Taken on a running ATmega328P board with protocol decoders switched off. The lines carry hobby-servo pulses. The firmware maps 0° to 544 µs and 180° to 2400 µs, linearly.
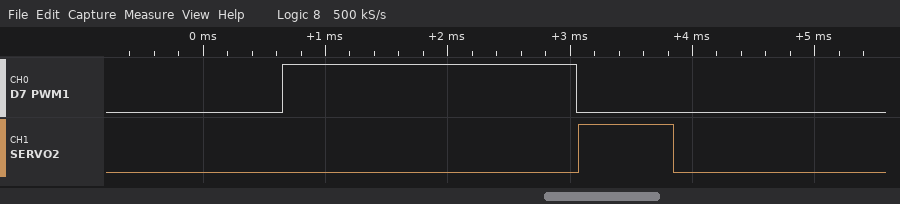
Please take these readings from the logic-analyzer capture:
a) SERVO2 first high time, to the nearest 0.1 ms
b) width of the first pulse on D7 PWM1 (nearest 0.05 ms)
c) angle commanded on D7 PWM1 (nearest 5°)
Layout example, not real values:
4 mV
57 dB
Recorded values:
0.8 ms
2.40 ms
180°
